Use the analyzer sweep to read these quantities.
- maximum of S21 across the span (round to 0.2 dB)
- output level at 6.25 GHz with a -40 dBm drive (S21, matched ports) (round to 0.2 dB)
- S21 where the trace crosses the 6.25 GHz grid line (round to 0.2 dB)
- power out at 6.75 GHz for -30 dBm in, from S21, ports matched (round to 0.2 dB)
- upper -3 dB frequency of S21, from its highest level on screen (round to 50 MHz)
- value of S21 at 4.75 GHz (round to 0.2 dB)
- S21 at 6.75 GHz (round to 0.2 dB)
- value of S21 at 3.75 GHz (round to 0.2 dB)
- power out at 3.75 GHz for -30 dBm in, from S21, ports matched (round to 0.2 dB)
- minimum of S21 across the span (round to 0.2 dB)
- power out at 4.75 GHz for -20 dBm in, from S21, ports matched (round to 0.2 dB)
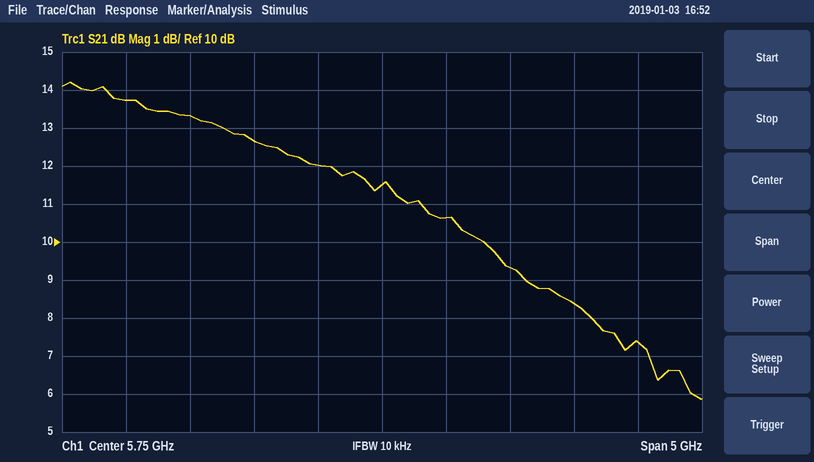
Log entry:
14.2 dB
-29.4 dBm
10.6 dB
-20.6 dBm
5.85 GHz
12.6 dB
9.4 dB
13.8 dB
-16.2 dBm
5.8 dB
-7.4 dBm
